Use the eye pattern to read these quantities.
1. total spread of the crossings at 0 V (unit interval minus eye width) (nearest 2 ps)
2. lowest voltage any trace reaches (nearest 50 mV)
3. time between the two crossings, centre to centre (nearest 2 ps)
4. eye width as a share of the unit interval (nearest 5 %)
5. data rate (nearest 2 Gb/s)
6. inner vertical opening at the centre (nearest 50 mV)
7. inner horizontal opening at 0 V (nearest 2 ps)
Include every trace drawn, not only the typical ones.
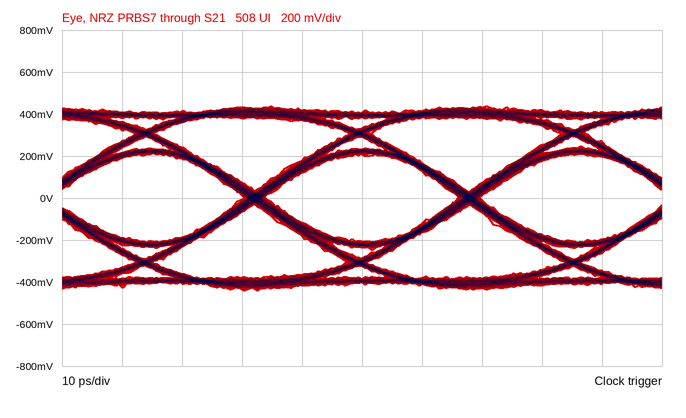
4 ps
-450 mV
36 ps
90 %
28 Gb/s
400 mV
32 ps
